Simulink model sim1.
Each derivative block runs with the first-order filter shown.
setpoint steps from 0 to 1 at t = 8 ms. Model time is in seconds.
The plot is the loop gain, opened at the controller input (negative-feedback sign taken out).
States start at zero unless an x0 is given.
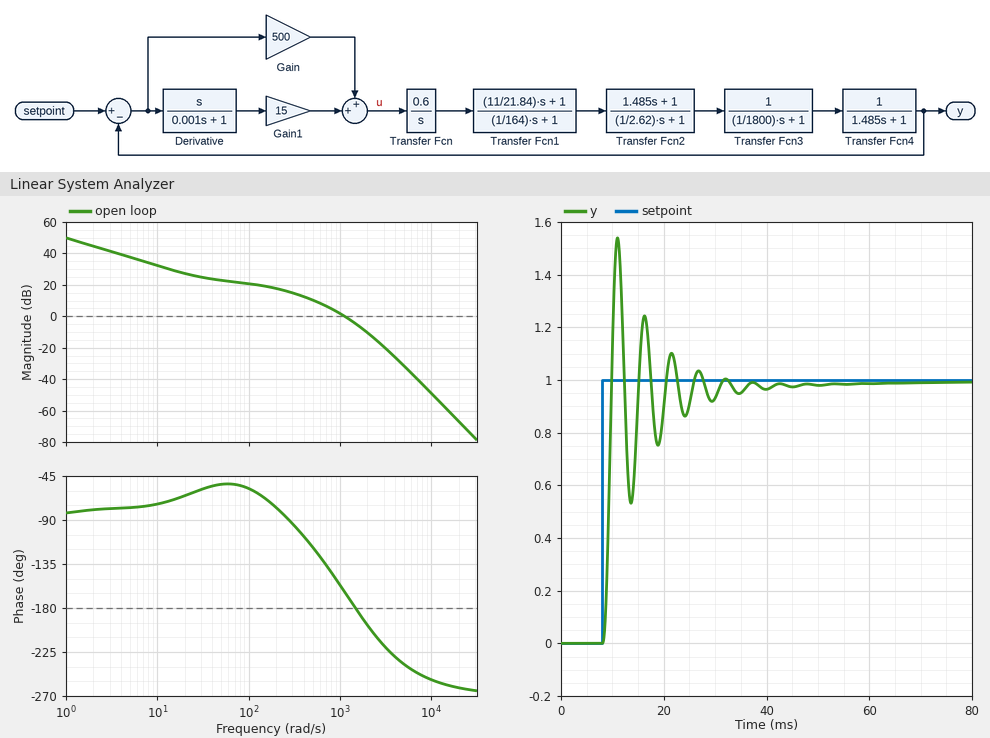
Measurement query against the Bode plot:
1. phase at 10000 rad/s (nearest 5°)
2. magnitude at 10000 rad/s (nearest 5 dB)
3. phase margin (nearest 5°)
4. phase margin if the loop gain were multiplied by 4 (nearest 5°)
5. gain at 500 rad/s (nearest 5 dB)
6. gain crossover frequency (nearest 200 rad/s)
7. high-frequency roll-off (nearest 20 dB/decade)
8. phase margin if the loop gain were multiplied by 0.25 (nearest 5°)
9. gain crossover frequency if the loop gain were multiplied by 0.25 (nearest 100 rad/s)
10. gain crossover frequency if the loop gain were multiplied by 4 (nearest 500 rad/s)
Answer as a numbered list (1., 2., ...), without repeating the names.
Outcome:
1. -255°
2. -50 dB
3. 15°
4. -20°
5. 10 dB
6. 1200 rad/s
7. -60 dB/decade
8. 70°
9. 400 rad/s
10. 2000 rad/s
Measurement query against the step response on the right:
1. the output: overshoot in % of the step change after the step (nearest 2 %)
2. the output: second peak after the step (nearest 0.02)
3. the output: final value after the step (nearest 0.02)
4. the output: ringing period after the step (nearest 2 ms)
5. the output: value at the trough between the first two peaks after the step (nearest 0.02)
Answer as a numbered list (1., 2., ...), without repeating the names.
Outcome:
1. 54 %
2. 1.24
3. 1.00
4. 6 ms
5. 0.54
